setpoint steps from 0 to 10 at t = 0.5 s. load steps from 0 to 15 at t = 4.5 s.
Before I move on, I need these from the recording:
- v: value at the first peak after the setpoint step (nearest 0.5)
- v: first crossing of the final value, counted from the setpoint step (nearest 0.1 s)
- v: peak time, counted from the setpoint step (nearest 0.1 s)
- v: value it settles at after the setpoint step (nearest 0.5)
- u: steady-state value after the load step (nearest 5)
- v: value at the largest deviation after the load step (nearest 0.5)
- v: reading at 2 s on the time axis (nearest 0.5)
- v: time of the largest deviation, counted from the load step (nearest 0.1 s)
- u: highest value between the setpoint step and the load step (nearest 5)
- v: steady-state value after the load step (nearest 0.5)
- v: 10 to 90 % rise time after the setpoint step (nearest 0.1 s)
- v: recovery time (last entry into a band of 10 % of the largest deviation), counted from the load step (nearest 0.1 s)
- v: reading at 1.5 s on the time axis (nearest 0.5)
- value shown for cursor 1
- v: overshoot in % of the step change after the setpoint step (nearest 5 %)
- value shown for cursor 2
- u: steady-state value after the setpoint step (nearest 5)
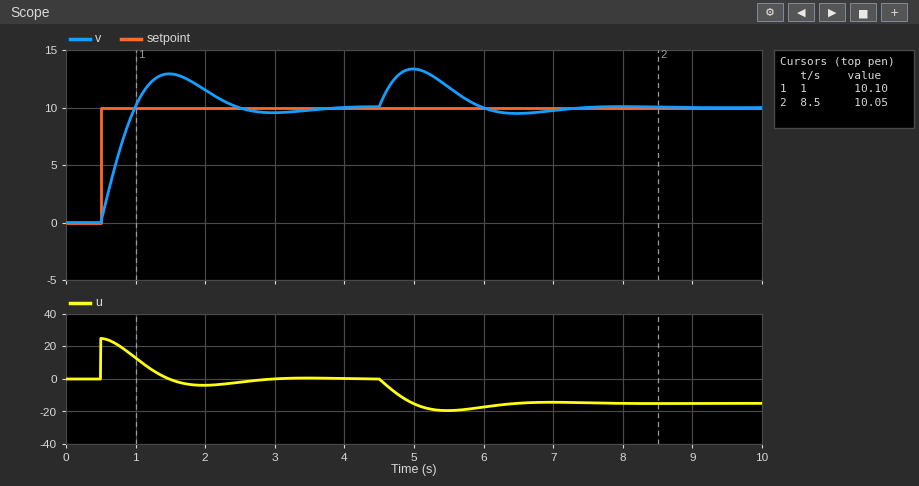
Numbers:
13.0
0.5 s
1.0 s
10.0
-15
13.5
11.5
0.5 s
25
10.0
0.4 s
2.4 s
13.0
10.10
30 %
10.05
0
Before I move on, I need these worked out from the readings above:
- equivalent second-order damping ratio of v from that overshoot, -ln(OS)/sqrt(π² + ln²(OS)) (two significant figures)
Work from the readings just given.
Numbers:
0.36
